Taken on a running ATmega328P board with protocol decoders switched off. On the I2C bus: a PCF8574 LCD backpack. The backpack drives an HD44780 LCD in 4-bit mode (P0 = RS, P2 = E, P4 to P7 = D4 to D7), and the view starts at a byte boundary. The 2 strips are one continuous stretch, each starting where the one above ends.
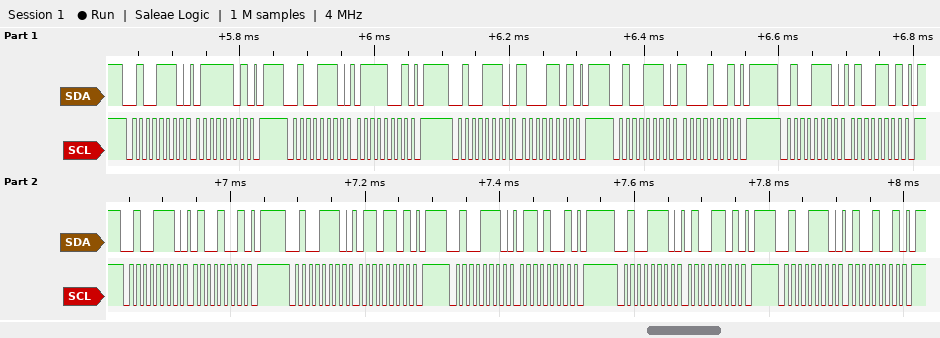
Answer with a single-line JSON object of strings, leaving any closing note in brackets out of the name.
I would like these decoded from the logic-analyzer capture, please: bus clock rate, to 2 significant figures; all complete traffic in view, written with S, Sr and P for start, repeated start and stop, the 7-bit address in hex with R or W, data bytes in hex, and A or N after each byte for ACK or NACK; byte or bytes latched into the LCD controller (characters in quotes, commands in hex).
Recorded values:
{"bus clock rate, to 2 significant figures": "100 kHz", "all complete traffic in view, written with S, Sr and P for start, repeated start and stop, the 7-bit address in hex with R or W, data bytes in hex, and A or N after each byte for ACK or NACK": "S 27W A 7D A P S 27W A 79 A P S 27W A 8D A P S 27W A 89 A P S 27W A 4D A P S 27W A 49 A P S 27W A 6D A P S 27W A 69 A P S 27W A 4D A P S 27W A 49 A P", "byte or bytes latched into the LCD controller": "'x' 'F'"}
